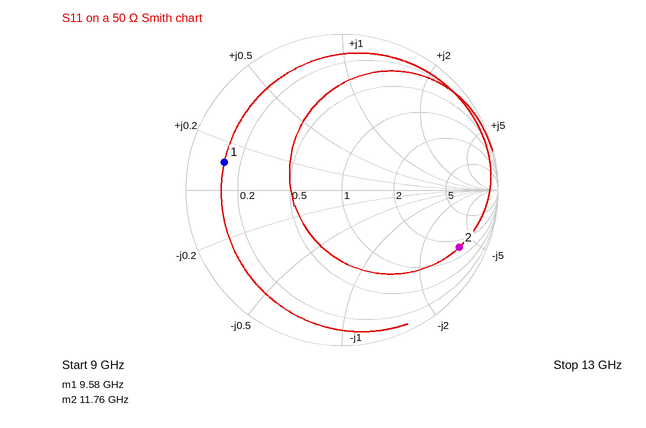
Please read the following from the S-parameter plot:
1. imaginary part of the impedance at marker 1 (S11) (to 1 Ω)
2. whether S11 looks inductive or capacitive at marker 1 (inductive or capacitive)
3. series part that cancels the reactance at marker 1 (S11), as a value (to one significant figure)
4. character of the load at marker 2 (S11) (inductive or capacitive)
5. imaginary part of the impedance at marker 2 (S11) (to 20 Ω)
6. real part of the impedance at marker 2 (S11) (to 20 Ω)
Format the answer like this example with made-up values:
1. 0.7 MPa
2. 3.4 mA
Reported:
1. +6 Ω
2. inductive
3. 3 pF
4. capacitive
5. -180 Ω
6. 80 Ω
